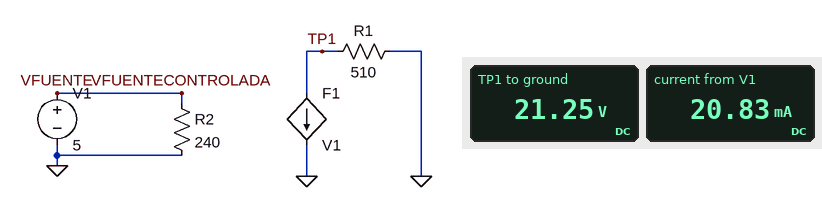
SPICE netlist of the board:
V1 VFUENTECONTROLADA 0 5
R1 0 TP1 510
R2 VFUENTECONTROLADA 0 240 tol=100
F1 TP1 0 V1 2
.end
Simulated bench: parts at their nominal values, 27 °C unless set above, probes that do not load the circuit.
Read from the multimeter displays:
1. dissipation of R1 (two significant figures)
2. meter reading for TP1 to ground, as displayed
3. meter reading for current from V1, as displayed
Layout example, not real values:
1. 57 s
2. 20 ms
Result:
1. 890 mW
2. 21.25 V
3. 20.83 mA
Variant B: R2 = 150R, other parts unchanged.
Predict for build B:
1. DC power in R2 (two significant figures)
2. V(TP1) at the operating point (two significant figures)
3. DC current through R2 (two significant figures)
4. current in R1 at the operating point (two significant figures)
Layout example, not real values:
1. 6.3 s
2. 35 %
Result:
1. 170 mW
2. 34 V
3. 33 mA
4. 67 mA
